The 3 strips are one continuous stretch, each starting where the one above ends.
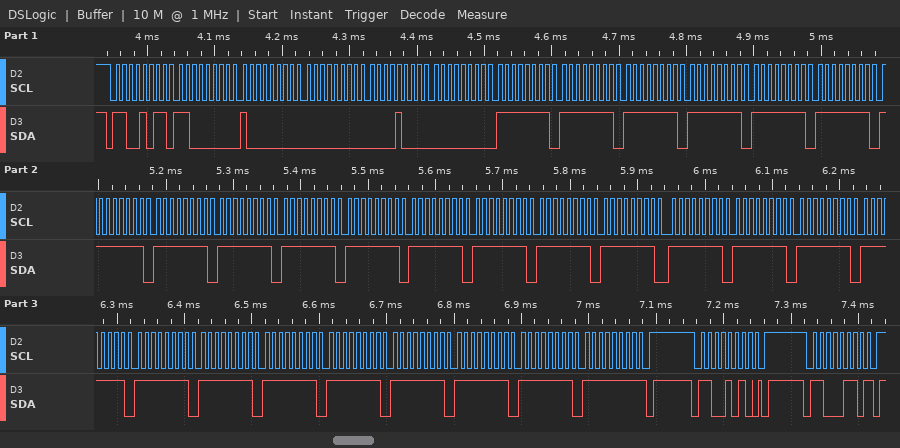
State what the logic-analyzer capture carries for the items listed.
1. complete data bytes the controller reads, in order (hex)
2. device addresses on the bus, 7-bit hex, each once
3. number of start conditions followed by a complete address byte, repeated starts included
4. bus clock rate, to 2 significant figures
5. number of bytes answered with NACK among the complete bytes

C0 80 00 08 00 FF FF FF FF FF FF FF FF FF FF FF FF FF FF FF FF FF FF FF FF FF FF FF FF FF FF FF
0x65 0x63
3
100 kHz
2
